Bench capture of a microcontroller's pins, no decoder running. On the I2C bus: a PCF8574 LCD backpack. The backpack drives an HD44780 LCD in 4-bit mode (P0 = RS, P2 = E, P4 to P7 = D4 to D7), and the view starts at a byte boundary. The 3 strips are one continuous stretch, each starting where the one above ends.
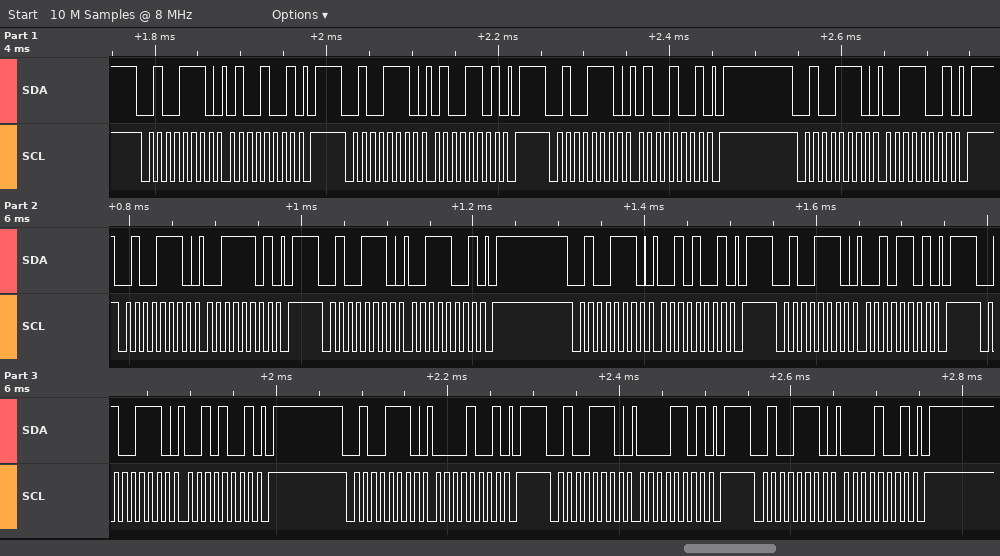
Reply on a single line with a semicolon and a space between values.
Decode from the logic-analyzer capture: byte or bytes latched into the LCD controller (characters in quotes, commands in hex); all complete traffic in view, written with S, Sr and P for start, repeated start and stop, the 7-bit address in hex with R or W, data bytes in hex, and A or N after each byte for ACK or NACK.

'C' ' '; S 27W A 49 A P S 27W A 4D A P S 27W A 49 A P S 27W A 39 A P S 27W A 3D A P S 27W A 39 A P S 27W A 29 A P S 27W A 2D A P S 27W A 29 A P S 27W A 09 A P S 27W A 0D A P S 27W A 09 A P
